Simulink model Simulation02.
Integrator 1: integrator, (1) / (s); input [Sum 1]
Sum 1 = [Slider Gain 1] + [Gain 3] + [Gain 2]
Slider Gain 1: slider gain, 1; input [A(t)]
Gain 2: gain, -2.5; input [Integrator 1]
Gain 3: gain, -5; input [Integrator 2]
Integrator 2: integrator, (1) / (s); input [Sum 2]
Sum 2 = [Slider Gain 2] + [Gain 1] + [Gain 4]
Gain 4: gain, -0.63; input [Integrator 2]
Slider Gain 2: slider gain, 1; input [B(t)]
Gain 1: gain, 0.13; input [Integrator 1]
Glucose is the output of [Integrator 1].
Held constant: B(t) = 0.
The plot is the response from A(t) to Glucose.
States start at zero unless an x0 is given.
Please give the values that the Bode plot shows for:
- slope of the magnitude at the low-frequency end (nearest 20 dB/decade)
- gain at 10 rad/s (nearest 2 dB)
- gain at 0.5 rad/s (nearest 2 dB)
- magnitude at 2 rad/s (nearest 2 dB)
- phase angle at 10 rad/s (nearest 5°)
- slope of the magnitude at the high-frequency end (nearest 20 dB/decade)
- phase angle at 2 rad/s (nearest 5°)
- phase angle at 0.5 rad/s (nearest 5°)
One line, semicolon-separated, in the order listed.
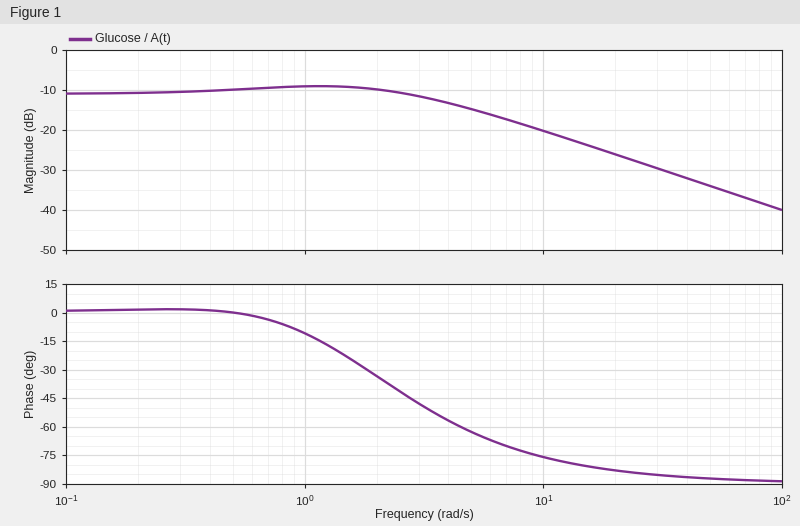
0 dB/decade; -20 dB; -10 dB; -10 dB; -75°; -20 dB/decade; -35°; 0°
